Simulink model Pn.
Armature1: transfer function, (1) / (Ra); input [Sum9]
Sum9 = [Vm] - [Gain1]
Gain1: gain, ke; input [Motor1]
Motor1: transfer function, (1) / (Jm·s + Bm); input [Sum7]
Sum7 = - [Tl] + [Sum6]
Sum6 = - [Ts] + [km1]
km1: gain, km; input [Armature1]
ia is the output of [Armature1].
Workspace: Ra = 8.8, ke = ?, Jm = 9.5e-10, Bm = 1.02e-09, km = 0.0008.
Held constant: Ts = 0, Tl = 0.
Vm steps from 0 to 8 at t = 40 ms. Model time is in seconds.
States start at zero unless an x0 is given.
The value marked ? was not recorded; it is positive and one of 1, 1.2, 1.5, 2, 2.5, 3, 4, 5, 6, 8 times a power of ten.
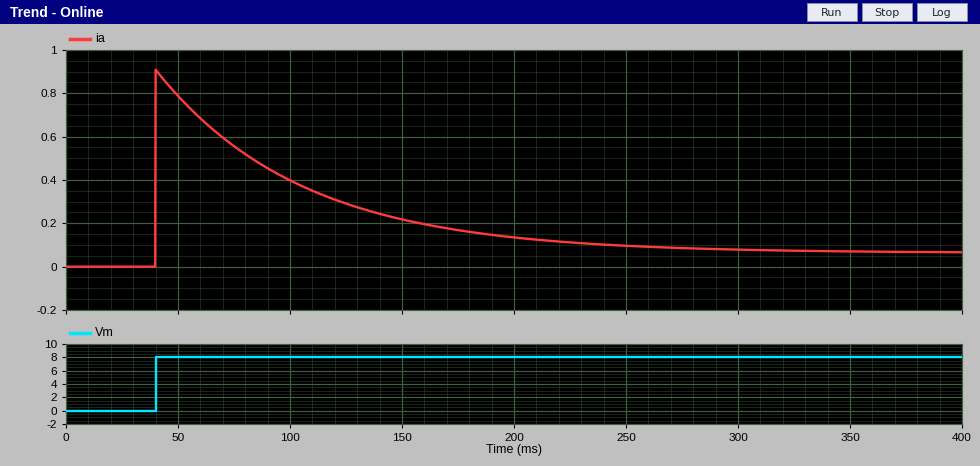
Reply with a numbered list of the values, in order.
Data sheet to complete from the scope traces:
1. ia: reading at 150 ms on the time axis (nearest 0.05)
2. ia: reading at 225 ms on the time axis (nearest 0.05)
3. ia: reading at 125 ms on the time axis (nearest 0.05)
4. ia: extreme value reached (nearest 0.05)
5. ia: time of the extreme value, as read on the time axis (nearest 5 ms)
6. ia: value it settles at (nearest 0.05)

1. 0.20
2. 0.10
3. 0.30
4. 0.90
5. 40 ms
6. 0.05
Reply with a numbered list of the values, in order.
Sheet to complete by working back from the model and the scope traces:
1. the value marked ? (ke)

1. 0.00015
